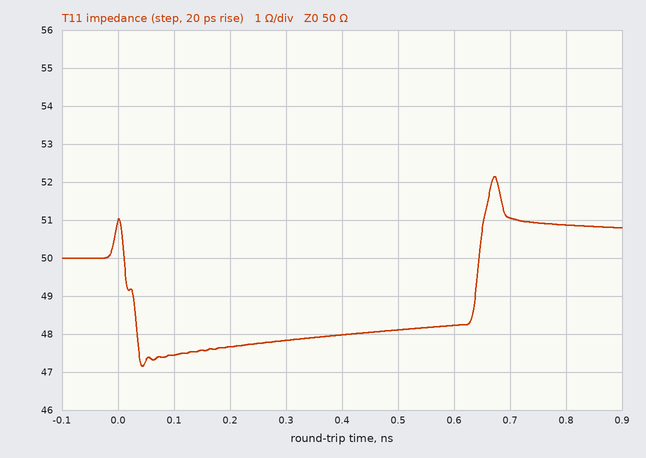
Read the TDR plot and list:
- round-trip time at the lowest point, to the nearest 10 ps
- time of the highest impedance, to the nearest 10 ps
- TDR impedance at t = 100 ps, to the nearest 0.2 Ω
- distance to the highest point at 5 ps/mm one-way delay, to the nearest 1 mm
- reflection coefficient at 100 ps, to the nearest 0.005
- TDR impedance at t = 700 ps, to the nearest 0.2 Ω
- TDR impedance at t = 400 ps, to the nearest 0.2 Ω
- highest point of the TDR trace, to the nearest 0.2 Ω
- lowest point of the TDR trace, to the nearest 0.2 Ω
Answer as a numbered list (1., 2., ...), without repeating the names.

1. 40 ps
2. 670 ps
3. 47.4 Ω
4. 67 mm
5. -0.025
6. 51.0 Ω
7. 48.0 Ω
8. 52.2 Ω
9. 47.2 Ω
